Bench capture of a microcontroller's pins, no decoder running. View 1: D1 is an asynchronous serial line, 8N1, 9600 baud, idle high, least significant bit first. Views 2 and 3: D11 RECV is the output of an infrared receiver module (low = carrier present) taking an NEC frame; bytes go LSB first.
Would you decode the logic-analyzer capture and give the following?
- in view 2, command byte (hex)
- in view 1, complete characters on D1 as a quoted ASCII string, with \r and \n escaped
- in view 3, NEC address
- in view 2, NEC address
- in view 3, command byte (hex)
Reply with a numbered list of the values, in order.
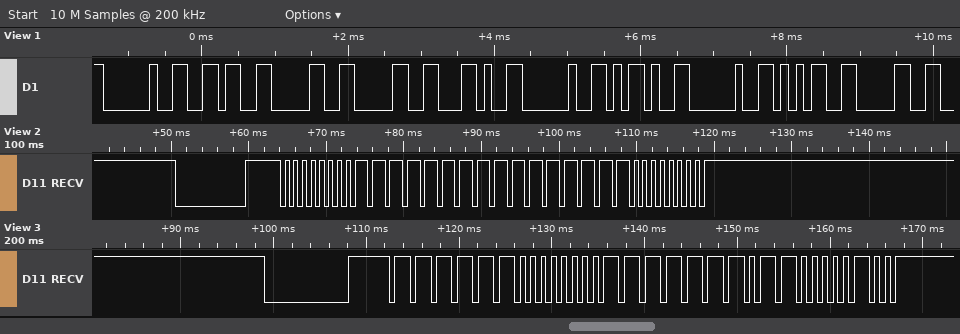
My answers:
1. 0xFF
2. " 600, - 50"
3. 0x3F
4. 0x00
5. 0xDF
